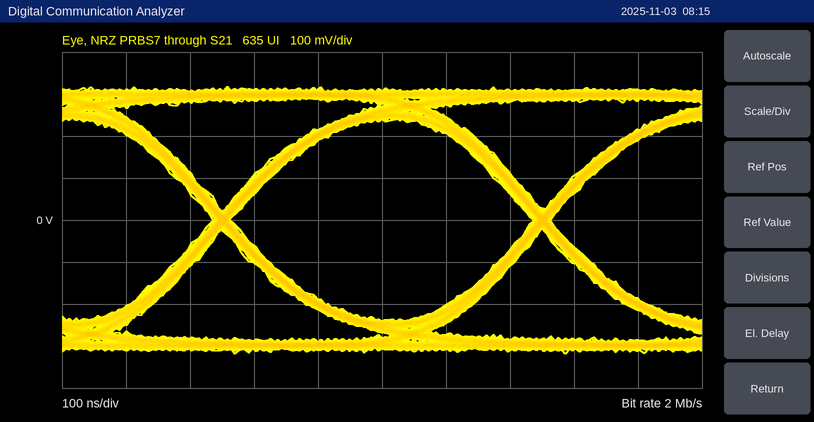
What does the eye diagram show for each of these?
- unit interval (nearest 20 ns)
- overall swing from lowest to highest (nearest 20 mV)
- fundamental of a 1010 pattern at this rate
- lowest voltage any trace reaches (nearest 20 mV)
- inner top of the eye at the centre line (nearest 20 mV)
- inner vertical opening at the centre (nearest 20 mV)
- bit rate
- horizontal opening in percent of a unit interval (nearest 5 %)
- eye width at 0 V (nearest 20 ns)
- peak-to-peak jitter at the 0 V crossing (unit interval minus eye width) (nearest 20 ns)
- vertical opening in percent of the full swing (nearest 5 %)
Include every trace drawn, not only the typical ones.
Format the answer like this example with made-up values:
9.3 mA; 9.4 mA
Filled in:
500 ns; 640 mV; 1 MHz; -320 mV; 240 mV; 480 mV; 2 Mb/s; 95 %; 480 ns; 20 ns; 75 %
